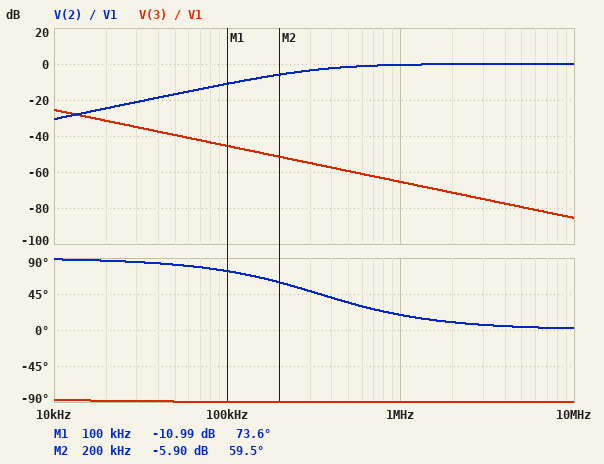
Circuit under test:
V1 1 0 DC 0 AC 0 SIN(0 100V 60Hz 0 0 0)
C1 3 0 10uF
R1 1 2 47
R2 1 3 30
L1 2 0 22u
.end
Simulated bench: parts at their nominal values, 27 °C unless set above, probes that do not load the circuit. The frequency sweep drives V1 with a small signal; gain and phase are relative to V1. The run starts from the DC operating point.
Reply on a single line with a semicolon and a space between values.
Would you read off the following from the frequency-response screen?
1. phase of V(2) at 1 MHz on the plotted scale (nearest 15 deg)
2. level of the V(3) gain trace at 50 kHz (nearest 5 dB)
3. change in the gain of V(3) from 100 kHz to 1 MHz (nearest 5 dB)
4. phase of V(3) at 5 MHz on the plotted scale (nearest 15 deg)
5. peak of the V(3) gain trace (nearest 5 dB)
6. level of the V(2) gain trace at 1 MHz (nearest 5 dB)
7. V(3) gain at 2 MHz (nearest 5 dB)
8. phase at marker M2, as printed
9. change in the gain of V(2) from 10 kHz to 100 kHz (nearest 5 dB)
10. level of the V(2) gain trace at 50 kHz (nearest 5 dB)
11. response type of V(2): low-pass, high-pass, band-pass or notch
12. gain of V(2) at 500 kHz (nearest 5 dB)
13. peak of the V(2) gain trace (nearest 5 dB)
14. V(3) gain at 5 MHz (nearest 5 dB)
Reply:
15 deg; -40 dB; -20 dB; -90 deg; -25 dB; 0 dB; -70 dB; 59.5 deg; 20 dB; -15 dB; high-pass; 0 dB; 0 dB; -80 dB
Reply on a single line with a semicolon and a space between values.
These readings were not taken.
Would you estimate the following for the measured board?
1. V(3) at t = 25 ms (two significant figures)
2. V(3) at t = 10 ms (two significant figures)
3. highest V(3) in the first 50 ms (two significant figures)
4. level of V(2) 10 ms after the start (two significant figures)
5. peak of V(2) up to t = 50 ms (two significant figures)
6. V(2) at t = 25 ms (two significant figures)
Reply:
11 V; -49 V; 99 V; -14 mV; 18 mV; -18 mV
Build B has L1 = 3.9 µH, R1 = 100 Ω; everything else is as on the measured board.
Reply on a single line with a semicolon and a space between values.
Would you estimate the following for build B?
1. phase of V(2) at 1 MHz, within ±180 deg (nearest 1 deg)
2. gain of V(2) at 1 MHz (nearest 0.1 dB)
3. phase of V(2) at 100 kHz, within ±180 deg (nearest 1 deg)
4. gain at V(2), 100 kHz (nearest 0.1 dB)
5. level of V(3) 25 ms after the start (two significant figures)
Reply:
76 deg; -12.5 dB; 89 deg; -32.2 dB; 11 V
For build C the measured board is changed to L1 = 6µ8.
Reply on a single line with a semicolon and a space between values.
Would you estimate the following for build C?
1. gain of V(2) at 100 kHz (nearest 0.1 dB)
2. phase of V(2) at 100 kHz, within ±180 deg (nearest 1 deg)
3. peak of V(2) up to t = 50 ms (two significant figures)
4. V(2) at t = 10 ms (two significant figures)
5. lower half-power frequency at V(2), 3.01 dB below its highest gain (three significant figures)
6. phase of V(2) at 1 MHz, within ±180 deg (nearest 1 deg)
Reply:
-20.9 dB; 85 deg; 5.5 mV; -4.4 mV; 1.10 MHz; 48 deg
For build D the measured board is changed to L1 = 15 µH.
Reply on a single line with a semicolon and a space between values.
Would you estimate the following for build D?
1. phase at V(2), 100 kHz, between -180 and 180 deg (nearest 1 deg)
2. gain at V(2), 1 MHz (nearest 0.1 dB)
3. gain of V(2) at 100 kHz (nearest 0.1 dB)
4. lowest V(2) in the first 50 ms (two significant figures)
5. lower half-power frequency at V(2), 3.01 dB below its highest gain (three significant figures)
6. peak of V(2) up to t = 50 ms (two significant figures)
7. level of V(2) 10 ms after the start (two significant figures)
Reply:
79 deg; -1.0 dB; -14.1 dB; -12 mV; 499 kHz; 12 mV; -9.7 mV
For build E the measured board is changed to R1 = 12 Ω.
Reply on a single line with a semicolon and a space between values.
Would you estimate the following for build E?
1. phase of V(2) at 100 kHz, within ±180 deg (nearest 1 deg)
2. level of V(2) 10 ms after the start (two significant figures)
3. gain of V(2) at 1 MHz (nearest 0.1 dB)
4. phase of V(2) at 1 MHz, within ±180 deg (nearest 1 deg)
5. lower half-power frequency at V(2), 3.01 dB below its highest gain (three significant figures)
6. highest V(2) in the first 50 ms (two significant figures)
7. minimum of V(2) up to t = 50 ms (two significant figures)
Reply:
41 deg; -56 mV; 0 dB; 5 deg; 86.8 kHz; 69 mV; -69 mV
